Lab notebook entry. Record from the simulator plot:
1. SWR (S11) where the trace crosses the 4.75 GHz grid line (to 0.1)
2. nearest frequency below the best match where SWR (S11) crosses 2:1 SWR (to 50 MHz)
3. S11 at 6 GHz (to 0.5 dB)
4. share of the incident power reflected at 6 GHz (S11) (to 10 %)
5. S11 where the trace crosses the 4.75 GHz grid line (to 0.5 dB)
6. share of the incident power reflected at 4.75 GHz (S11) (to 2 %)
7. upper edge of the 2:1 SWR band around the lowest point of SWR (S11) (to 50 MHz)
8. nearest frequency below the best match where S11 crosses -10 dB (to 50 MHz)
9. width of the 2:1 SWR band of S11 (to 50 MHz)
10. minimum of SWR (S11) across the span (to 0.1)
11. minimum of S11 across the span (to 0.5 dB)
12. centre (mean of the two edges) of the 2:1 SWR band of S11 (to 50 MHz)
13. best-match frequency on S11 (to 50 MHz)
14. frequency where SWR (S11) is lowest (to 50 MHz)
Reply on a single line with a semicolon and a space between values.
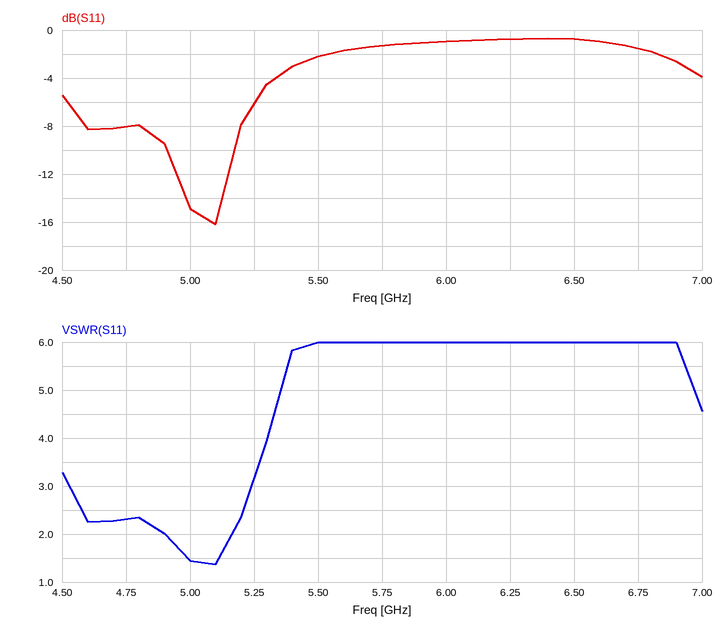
2.3; 4.90 GHz; -1.0 dB; 80 %; -8.0 dB; 16 %; 5.15 GHz; 4.90 GHz; 250 MHz; 1.4; -16.0 dB; 5.05 GHz; 5.10 GHz; 5.10 GHz
